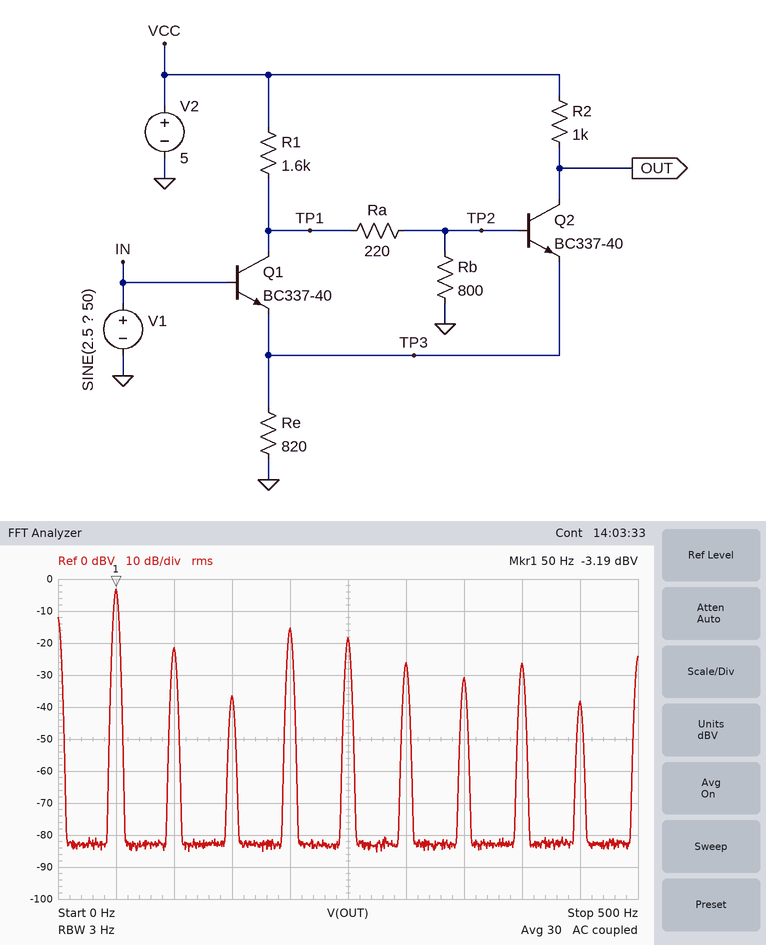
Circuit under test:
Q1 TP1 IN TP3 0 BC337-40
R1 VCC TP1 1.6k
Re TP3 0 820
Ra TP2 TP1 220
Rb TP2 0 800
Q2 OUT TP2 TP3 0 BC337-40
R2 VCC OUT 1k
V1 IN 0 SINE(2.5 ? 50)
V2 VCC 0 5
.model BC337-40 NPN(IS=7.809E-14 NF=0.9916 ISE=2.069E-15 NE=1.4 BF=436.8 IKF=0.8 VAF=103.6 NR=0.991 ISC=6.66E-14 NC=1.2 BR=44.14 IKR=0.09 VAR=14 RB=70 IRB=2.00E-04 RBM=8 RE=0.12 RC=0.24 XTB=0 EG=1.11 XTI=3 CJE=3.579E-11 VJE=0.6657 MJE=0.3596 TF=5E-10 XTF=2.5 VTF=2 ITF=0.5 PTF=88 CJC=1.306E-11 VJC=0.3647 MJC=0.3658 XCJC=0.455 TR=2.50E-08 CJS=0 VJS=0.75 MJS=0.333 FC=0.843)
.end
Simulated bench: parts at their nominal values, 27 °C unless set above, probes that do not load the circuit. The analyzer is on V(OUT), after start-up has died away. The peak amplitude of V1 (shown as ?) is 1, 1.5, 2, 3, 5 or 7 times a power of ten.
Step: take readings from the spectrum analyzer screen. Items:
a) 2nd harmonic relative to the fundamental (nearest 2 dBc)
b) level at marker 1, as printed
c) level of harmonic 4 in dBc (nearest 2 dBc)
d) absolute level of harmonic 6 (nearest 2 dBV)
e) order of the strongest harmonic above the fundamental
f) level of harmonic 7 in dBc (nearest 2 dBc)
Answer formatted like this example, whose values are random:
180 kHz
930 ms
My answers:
-18 dBc
-3.19 dBV
-12 dBc
-26 dBV
4
-28 dBc
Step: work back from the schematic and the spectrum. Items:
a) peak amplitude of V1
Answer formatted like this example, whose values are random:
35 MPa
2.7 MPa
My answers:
7 V
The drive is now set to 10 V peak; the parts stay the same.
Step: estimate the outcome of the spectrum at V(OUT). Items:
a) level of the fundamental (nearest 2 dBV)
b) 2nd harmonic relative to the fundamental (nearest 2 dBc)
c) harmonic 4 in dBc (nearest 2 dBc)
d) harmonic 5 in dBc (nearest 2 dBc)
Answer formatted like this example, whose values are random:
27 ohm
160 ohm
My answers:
2 dBV
-8 dBc
-18 dBc
-28 dBc
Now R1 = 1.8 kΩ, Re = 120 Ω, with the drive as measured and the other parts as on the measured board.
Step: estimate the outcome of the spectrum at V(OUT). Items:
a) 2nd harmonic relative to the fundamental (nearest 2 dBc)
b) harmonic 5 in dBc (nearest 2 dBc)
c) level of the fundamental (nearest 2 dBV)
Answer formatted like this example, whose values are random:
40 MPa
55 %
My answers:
-16 dBc
-20 dBc
6 dBV
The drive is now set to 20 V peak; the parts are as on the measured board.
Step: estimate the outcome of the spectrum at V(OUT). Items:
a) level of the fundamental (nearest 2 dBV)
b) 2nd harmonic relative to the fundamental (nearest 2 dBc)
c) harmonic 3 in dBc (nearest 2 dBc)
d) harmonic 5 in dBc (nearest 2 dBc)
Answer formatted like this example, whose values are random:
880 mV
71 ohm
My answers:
12 dBV
-6 dBc
-20 dBc
-28 dBc
